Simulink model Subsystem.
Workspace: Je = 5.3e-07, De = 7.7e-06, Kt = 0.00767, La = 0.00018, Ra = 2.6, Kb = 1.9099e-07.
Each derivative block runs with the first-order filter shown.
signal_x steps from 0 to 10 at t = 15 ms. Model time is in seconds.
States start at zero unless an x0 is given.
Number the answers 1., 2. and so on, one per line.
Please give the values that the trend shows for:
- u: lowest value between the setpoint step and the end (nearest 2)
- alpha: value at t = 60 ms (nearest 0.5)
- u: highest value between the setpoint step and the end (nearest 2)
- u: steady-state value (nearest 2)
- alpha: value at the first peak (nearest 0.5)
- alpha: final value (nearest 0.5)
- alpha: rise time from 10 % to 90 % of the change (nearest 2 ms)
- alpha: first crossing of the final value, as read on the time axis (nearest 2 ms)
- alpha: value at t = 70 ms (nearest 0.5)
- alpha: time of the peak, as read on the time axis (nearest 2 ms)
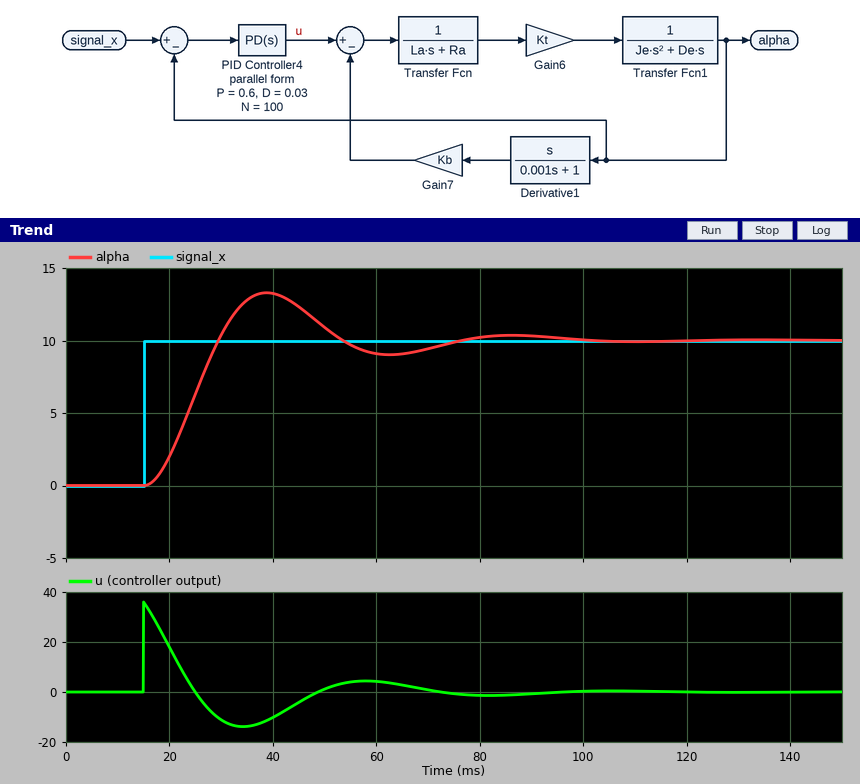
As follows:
1. -14
2. 9.0
3. 36
4. 0
5. 13.5
6. 10.0
7. 10 ms
8. 30 ms
9. 9.5
10. 38 ms
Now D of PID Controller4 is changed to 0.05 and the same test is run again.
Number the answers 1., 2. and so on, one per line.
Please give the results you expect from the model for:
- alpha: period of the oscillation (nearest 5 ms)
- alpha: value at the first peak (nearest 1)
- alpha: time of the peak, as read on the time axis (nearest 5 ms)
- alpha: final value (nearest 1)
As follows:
1. 35 ms
2. 14
3. 35 ms
4. 10
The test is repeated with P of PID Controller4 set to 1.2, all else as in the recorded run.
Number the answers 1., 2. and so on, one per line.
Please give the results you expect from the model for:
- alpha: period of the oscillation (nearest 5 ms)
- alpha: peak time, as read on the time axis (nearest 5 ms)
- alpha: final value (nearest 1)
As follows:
1. 45 ms
2. 35 ms
3. 10
